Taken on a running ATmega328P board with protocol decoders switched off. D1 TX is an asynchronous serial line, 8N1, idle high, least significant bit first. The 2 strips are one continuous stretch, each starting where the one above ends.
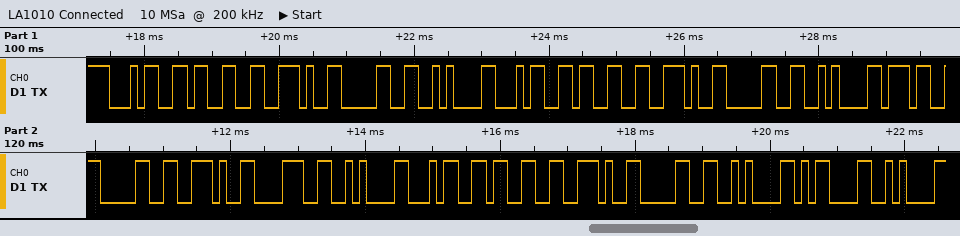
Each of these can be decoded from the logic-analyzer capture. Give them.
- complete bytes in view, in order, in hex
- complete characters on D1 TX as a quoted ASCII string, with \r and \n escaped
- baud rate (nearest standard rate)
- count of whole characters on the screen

0x34 0x33 0x2E 0x30 0x0A 0x34 0x33 0x2E 0x30 0x0A 0x37 0x30 0x2E 0x38 0x0A 0x34 0x33 0x2E 0x30 0x0A 0x0D 0x0A
"43.0\n43.0\n70.8\n43.0\n\r\n"
9600 baud
22
